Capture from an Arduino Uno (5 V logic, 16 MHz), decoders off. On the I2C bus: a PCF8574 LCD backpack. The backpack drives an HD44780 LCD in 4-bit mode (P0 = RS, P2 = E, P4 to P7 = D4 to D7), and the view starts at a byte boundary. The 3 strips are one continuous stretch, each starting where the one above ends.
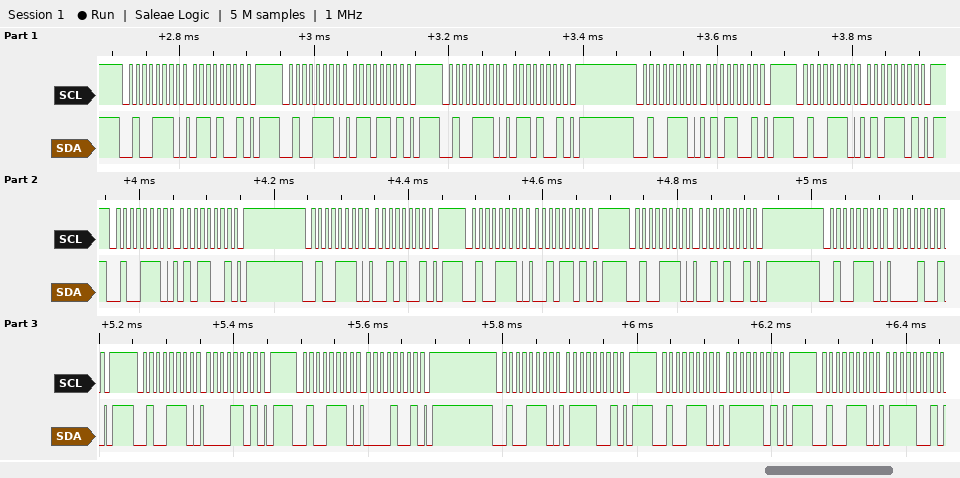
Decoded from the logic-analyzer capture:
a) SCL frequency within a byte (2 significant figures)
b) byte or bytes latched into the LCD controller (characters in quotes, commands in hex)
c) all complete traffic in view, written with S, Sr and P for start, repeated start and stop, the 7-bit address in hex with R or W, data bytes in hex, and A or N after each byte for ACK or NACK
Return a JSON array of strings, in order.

["100 kHz", "'e' ' '", "S 27W A 69 A P S 27W A 6D A P S 27W A 69 A P S 27W A 59 A P S 27W A 5D A P S 27W A 59 A P S 27W A 29 A P S 27W A 2D A P S 27W A 29 A P S 27W A 09 A P S 27W A 0D A P S 27W A 09 A P S 27W A 79 A P S 27W A 7D A P S 27W A 79 A"]
